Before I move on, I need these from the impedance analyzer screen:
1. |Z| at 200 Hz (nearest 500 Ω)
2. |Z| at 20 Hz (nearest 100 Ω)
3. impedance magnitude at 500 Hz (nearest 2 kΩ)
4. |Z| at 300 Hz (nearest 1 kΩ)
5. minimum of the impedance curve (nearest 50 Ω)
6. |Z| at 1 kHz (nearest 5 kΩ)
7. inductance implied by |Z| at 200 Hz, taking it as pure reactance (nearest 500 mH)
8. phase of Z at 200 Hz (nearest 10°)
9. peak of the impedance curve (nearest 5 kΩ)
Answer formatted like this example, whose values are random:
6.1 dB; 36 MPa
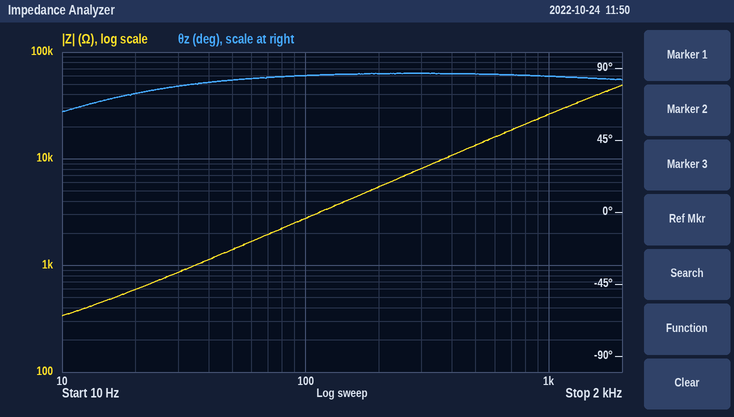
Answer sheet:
5.5 kΩ; 600 Ω; 14 kΩ; 8 kΩ; 350 Ω; 25 kΩ; 4.5 H; 90°; 50 kΩ
